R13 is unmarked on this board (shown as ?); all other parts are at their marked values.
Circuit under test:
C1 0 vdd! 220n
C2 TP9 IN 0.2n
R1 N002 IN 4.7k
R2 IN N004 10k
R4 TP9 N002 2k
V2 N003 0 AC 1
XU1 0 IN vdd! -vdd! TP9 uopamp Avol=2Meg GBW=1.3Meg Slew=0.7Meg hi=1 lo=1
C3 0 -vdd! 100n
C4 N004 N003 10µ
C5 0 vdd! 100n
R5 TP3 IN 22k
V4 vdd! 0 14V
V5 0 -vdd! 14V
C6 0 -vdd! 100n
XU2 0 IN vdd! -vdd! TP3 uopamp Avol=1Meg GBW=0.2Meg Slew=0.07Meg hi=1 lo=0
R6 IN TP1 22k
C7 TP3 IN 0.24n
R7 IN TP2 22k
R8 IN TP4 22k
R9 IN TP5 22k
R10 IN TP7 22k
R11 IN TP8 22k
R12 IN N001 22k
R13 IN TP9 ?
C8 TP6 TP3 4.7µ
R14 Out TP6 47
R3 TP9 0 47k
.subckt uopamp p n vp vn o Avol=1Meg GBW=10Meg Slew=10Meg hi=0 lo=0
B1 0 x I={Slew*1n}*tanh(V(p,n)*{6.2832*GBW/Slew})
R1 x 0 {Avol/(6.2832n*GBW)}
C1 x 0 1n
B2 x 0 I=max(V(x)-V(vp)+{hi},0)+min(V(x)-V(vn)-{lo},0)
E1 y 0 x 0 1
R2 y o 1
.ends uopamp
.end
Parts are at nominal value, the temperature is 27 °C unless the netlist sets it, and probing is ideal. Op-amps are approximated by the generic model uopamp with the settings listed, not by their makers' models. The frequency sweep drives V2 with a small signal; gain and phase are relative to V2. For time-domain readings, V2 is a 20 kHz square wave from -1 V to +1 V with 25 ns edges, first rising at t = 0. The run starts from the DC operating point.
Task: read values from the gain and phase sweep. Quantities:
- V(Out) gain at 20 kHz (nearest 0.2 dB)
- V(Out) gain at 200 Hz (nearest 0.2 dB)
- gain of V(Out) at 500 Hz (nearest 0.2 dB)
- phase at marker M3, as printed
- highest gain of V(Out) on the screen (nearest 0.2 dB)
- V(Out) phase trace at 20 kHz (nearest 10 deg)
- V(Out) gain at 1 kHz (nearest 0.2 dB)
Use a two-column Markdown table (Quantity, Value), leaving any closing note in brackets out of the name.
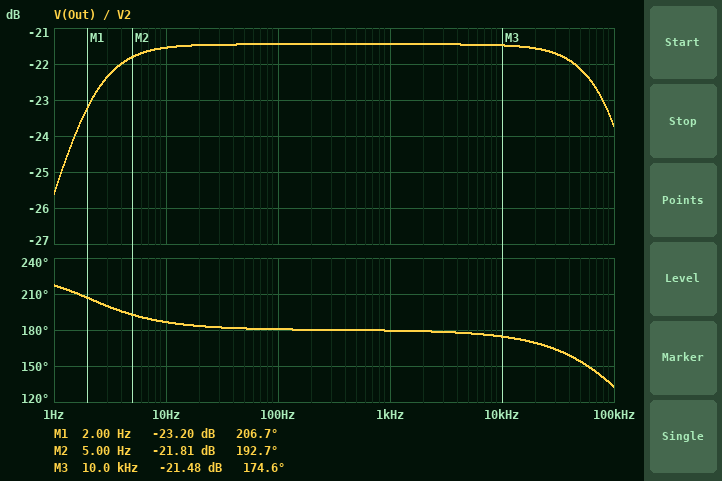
| Quantity | Value |
|---|---|
| V(Out) gain at 20 kHz | -21.6 dB |
| V(Out) gain at 200 Hz | -21.4 dB |
| gain of V(Out) at 500 Hz | -21.4 dB |
| phase at marker M3, as printed | 174.6 deg |
| highest gain of V(Out) on the screen | -21.4 dB |
| V(Out) phase trace at 20 kHz | 170 deg |
| V(Out) gain at 1 kHz | -21.4 dB |
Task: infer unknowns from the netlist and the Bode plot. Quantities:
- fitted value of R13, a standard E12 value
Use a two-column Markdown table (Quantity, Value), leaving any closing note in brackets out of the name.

| Quantity | Value |
|---|---|
| fitted value of R13, a standard E12 value | 39 kΩ |
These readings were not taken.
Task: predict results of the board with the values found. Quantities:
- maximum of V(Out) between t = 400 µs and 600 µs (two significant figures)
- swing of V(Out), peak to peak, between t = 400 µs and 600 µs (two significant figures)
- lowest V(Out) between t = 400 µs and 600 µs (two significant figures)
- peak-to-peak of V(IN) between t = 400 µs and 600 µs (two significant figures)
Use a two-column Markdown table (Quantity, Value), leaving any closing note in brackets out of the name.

| Quantity | Value |
|---|---|
| maximum of V(Out) between t = 400 µs and 600 µs | 82 mV |
| swing of V(Out), peak to peak, between t = 400 µs and 600 µs | 150 mV |
| lowest V(Out) between t = 400 µs and 600 µs | -66 mV |
| peak-to-peak of V(IN) between t = 400 µs and 600 µs | 180 mV |
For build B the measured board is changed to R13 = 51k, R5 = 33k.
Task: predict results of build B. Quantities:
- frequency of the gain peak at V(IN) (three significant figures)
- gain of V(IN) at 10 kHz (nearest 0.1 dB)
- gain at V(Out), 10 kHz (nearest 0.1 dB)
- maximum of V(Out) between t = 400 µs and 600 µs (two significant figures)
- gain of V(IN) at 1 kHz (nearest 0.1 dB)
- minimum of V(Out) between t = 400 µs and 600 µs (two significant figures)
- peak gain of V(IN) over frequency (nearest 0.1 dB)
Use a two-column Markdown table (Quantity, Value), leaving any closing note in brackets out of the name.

| Quantity | Value |
|---|---|
| frequency of the gain peak at V(IN) | 286 kHz |
| gain of V(IN) at 10 kHz | -47.1 dB |
| gain at V(Out), 10 kHz | -21.1 dB |
| maximum of V(Out) between t = 400 µs and 600 µs | 86 mV |
| gain of V(IN) at 1 kHz | -67.1 dB |
| minimum of V(Out) between t = 400 µs and 600 µs | -69 mV |
| peak gain of V(IN) over frequency | -27.0 dB |
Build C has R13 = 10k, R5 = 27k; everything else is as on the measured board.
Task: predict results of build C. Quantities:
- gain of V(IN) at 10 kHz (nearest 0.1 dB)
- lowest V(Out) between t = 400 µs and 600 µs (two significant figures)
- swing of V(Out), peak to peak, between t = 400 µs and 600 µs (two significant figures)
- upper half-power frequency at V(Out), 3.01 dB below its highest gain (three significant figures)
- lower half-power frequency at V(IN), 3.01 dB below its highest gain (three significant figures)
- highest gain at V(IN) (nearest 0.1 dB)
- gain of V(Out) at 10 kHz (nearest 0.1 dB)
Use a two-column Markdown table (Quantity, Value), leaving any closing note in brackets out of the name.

| Quantity | Value |
|---|---|
| gain of V(IN) at 10 kHz | -50.4 dB |
| lowest V(Out) between t = 400 µs and 600 µs | -48 mV |
| swing of V(Out), peak to peak, between t = 400 µs and 600 µs | 110 mV |
| upper half-power frequency at V(Out), 3.01 dB below its highest gain | 171 kHz |
| lower half-power frequency at V(IN), 3.01 dB below its highest gain | 124 kHz |
| highest gain at V(IN) | -27.3 dB |
| gain of V(Out) at 10 kHz | -24.4 dB |
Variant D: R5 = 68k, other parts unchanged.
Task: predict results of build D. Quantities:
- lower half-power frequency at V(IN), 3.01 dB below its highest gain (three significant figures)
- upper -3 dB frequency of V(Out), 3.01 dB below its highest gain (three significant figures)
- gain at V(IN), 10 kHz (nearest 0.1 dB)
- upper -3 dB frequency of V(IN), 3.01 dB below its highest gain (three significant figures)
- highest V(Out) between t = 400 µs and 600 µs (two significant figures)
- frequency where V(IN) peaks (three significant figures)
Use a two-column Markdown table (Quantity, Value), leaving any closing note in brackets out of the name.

| Quantity | Value |
|---|---|
| lower half-power frequency at V(IN), 3.01 dB below its highest gain | 92.8 kHz |
| upper -3 dB frequency of V(Out), 3.01 dB below its highest gain | 118 kHz |
| gain at V(IN), 10 kHz | -47.3 dB |
| upper -3 dB frequency of V(IN), 3.01 dB below its highest gain | 897 kHz |
| highest V(Out) between t = 400 µs and 600 µs | 84 mV |
| frequency where V(IN) peaks | 289 kHz |
